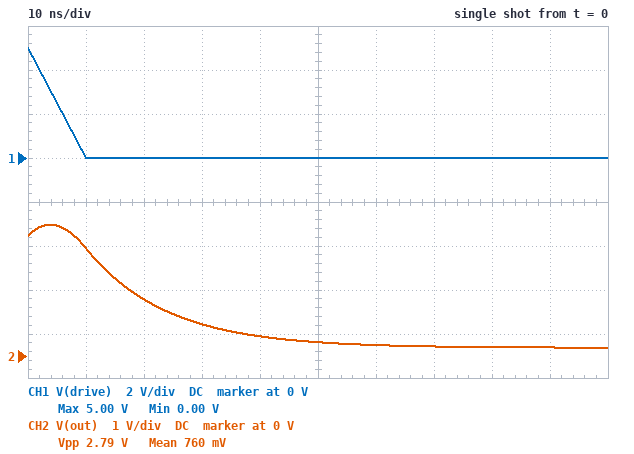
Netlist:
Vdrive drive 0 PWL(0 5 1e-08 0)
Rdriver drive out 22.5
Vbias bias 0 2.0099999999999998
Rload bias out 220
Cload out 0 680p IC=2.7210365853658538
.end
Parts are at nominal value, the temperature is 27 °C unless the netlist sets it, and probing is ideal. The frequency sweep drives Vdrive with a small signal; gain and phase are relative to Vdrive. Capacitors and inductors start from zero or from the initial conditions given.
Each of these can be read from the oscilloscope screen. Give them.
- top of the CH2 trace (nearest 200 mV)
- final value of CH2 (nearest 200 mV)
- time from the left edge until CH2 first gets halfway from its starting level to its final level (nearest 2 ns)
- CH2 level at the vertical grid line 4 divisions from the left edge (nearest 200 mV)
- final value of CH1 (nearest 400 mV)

3.0 V
200 mV
18 ns
400 mV
0 V
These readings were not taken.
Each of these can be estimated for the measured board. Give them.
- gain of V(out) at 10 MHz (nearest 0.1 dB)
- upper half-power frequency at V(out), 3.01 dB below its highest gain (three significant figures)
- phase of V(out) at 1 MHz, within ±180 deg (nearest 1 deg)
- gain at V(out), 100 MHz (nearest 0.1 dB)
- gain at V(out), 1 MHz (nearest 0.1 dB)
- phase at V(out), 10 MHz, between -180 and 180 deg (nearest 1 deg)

-3.3 dB
11.5 MHz
-5 deg
-19.7 dB
-0.9 dB
-41 deg
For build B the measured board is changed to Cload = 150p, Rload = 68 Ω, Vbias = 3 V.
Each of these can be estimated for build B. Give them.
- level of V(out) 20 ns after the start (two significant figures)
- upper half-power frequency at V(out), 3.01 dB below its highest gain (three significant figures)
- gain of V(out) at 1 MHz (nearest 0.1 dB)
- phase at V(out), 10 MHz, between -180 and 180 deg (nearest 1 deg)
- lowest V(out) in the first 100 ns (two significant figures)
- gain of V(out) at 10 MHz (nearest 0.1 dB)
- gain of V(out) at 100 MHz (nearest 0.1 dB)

760 mV
62.8 MHz
-2.5 dB
-9 deg
750 mV
-2.6 dB
-8.0 dB
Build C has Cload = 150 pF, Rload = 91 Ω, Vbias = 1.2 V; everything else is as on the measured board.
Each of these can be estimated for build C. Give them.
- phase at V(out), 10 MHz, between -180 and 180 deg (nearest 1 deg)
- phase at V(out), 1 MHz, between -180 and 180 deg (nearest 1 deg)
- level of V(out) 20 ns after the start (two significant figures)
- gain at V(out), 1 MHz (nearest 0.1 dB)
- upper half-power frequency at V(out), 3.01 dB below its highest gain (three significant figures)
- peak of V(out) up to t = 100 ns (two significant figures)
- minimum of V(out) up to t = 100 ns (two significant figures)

-10 deg
-1 deg
260 mV
-1.9 dB
58.8 MHz
3.3 V
240 mV
